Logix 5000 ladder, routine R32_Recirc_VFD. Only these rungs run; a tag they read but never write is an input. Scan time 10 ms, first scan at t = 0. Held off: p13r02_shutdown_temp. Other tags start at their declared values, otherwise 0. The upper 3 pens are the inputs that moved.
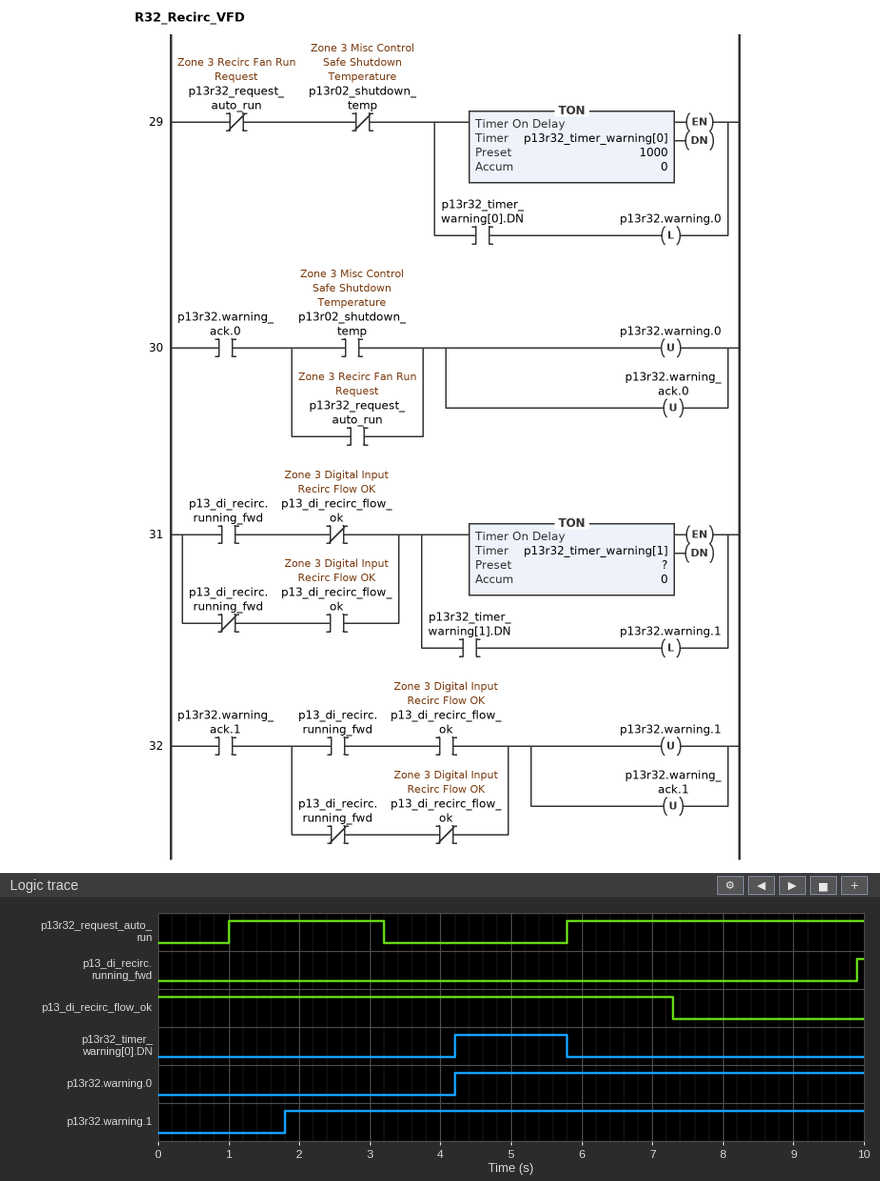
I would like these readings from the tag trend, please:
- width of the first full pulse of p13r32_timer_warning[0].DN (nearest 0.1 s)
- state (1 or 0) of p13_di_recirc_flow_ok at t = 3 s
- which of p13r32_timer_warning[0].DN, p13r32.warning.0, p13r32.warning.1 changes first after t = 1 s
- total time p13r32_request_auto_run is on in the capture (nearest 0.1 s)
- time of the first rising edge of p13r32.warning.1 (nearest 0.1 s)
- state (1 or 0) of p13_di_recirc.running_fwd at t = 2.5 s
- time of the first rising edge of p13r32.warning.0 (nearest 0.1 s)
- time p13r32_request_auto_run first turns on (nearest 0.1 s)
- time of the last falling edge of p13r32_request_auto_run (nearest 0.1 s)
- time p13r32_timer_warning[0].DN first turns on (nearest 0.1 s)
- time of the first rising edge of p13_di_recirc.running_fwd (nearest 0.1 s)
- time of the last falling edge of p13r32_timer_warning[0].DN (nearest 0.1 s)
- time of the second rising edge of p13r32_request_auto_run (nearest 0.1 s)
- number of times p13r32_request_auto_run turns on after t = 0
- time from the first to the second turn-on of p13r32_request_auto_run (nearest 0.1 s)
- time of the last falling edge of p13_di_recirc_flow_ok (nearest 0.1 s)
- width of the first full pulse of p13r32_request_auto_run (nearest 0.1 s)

1.6 s
1
p13r32.warning.1
6.4 s
1.8 s
0
4.2 s
1.0 s
3.2 s
4.2 s
9.9 s
5.8 s
5.8 s
2
4.8 s
7.3 s
2.2 s
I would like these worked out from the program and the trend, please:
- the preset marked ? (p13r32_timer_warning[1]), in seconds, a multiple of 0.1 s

1.8 s
